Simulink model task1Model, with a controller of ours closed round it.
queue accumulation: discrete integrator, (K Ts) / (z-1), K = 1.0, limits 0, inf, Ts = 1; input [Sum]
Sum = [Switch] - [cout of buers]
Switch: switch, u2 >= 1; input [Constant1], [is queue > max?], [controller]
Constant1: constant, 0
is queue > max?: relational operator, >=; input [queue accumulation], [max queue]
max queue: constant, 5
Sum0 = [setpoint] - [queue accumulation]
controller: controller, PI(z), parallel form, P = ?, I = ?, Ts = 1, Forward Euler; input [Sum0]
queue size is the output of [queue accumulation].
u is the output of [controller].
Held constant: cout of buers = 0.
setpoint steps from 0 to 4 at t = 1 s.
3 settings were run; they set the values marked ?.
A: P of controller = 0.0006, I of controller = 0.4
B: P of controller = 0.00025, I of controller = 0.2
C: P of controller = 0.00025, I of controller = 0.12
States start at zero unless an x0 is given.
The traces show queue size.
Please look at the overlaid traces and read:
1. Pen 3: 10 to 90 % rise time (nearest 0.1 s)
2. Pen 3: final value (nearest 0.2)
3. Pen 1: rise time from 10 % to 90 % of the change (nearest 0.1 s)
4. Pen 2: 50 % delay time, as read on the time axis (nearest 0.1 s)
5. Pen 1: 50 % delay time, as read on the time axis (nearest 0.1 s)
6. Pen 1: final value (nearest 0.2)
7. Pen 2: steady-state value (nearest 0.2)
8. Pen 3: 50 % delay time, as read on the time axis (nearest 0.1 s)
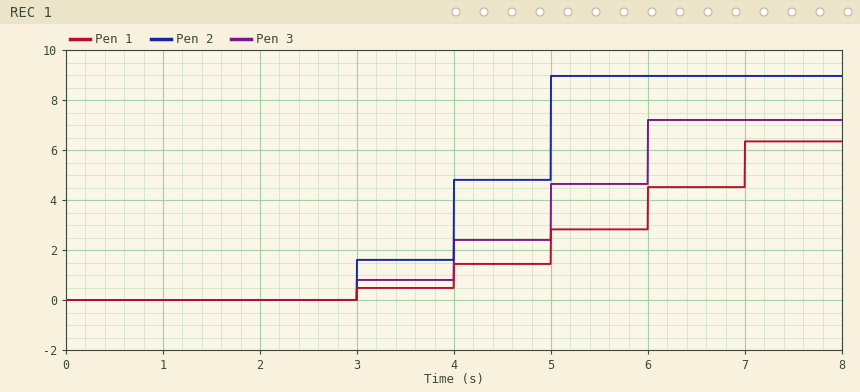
3.0 s
7.2
3.0 s
4.0 s
6.0 s
6.4
9.0
5.0 s
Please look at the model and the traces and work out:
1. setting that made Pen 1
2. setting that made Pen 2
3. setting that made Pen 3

C
A
B
